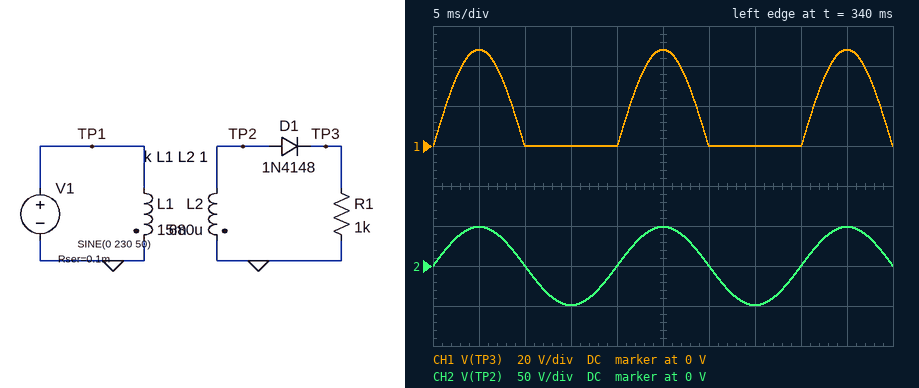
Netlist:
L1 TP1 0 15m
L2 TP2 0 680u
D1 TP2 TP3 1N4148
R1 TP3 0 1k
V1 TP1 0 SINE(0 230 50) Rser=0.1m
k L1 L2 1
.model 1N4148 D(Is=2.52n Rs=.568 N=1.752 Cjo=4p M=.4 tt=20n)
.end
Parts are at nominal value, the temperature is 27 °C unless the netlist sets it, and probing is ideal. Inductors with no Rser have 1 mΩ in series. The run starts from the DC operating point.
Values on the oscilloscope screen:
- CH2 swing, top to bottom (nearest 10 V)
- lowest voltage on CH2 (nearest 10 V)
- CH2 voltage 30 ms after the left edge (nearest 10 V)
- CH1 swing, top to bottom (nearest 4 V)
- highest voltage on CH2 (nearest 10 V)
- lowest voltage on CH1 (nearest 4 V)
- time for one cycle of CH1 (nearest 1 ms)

100 V
-50 V
0 V
48 V
50 V
0 V
20 ms
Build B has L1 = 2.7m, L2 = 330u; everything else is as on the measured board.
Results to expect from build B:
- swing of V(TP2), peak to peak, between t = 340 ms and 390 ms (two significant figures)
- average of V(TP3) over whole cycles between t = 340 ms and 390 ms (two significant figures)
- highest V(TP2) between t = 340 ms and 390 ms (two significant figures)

160 V
25 V
80 V
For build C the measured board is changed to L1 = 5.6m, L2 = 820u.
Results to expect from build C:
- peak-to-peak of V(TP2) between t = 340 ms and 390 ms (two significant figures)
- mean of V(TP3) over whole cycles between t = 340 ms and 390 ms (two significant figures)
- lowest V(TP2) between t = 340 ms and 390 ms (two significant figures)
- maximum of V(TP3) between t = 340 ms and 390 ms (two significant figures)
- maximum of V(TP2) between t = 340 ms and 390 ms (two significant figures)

180 V
28 V
-88 V
87 V
88 V
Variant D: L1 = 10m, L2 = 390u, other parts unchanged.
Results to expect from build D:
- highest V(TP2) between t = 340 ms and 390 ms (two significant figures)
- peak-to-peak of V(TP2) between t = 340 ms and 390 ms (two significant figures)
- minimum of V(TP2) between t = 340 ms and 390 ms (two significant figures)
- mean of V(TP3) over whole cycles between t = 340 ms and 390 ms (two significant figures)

45 V
91 V
-45 V
14 V
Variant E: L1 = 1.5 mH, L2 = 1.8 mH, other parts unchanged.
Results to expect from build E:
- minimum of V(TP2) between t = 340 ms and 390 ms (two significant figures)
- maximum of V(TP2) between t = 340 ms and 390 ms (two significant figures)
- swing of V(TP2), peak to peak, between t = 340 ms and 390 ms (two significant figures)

-250 V
250 V
500 V
